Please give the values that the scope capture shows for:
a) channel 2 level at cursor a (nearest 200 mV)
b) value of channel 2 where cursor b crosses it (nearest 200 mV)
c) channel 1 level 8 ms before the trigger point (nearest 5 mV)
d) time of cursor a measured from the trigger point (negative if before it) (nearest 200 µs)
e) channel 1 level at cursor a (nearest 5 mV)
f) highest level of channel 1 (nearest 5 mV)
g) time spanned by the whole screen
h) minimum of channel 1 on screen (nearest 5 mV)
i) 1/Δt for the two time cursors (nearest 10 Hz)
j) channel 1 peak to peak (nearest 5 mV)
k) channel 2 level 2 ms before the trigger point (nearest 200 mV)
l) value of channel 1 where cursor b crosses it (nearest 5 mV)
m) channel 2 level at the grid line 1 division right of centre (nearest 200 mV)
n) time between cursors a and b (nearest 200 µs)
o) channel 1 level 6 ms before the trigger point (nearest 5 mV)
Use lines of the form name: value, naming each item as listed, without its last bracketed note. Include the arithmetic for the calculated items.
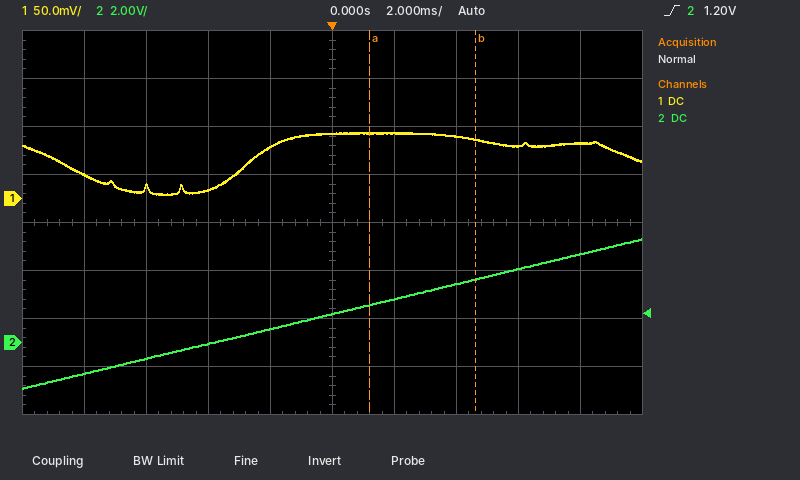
channel 2 level at cursor a: 1.6 V
value of channel 2 where cursor b crosses it: 2.6 V
channel 1 level 8 ms before the trigger point: 25 mV
time of cursor a measured from the trigger point (negative if before it): +1.2 ms
channel 1 level at cursor a: 70 mV
highest level of channel 1: 70 mV
time spanned by the whole screen: 20 ms
minimum of channel 1 on screen: 5 mV
1/Δt for the two time cursors: 1 / 3.4 ms ≈ 290 Hz
channel 1 peak to peak: 70 mV − (5 mV) = 65 mV
channel 2 level 2 ms before the trigger point: 600 mV
value of channel 1 where cursor b crosses it: 60 mV
channel 2 level at the grid line 1 division right of centre: 1.8 V
time between cursors a and b: 3.4 ms
channel 1 level 6 ms before the trigger point: 10 mV
